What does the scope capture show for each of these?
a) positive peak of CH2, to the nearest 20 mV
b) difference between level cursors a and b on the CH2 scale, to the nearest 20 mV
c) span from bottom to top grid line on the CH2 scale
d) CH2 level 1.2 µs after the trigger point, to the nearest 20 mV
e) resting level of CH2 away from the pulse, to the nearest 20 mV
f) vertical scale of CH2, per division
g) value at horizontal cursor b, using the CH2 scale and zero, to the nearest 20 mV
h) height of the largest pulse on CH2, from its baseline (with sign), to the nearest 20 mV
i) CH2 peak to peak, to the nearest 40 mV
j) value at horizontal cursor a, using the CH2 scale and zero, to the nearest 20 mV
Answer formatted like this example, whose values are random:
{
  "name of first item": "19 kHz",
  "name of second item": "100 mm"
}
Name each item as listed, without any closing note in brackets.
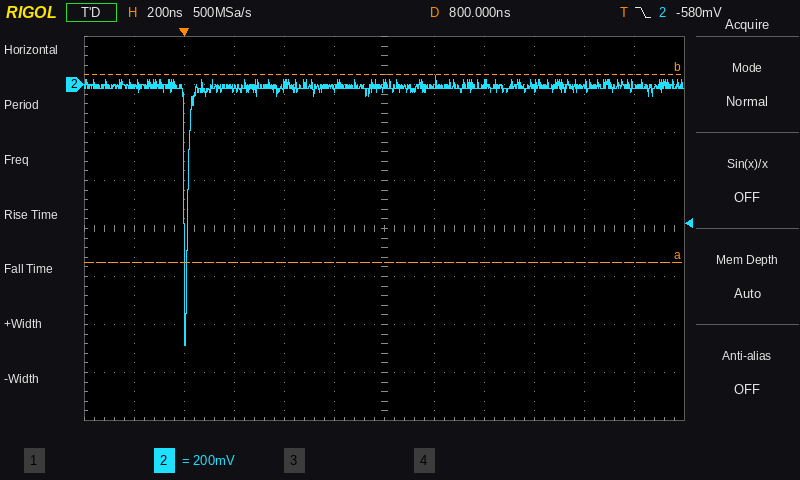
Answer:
{
  "positive peak of CH2, to the nearest 20 mV": "40 mV",
  "difference between level cursors a and b on the CH2 scale, to the nearest 20 mV": "780 mV",
  "span from bottom to top grid line on the CH2 scale": "1.6 V",
  "CH2 level 1.2 µs after the trigger point, to the nearest 20 mV": "0 mV",
  "resting level of CH2 away from the pulse, to the nearest 20 mV": "0 mV",
  "vertical scale of CH2, per division": "200 mV",
  "value at horizontal cursor b, using the CH2 scale and zero, to the nearest 20 mV": "40 mV",
  "height of the largest pulse on CH2, from its baseline (with sign), to the nearest 20 mV": "-1.08 V",
  "CH2 peak to peak, to the nearest 40 mV": "1.12 V",
  "value at horizontal cursor a, using the CH2 scale and zero, to the nearest 20 mV": "-740 mV"
}
